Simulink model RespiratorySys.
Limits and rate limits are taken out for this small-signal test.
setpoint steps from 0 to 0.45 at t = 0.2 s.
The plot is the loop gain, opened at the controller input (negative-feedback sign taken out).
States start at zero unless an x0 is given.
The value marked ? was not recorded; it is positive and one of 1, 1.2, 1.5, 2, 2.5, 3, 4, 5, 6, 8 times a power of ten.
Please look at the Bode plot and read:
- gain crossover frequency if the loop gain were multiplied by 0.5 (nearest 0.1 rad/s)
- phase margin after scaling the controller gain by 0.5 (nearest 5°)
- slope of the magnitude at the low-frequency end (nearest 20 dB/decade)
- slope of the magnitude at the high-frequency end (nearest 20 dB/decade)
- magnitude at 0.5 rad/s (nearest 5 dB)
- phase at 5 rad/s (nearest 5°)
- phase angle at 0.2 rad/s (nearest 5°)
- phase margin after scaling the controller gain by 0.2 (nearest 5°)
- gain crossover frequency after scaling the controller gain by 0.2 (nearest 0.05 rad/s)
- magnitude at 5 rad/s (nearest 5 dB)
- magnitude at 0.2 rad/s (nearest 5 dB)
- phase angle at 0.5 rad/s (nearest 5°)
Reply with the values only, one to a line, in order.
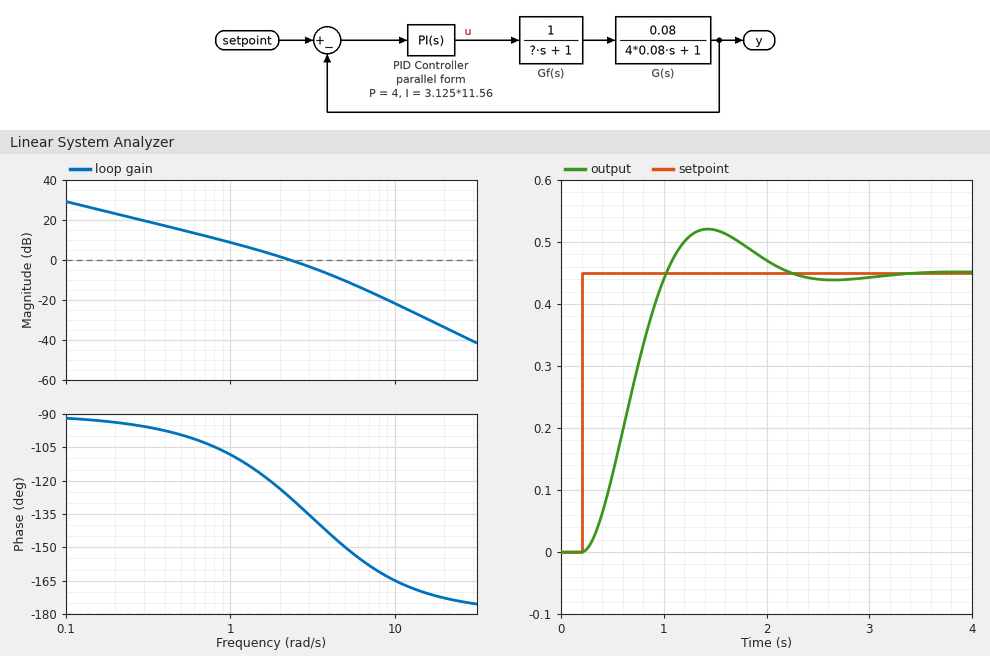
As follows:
1.3 rad/s
65°
-20 dB/decade
-40 dB/decade
15 dB
-150°
-95°
80°
0.55 rad/s
-10 dB
25 dB
-100°
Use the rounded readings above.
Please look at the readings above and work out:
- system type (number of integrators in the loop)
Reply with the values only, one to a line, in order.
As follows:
1
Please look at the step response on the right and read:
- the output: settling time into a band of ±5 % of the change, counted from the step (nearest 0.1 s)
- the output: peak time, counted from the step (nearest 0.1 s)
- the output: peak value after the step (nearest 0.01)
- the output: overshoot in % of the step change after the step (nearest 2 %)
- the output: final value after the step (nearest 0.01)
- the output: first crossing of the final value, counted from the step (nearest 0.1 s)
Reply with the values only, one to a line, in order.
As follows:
1.8 s
1.2 s
0.52
16 %
0.45
0.8 s
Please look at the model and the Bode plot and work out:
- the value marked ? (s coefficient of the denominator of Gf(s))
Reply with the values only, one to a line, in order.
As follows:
0.12
